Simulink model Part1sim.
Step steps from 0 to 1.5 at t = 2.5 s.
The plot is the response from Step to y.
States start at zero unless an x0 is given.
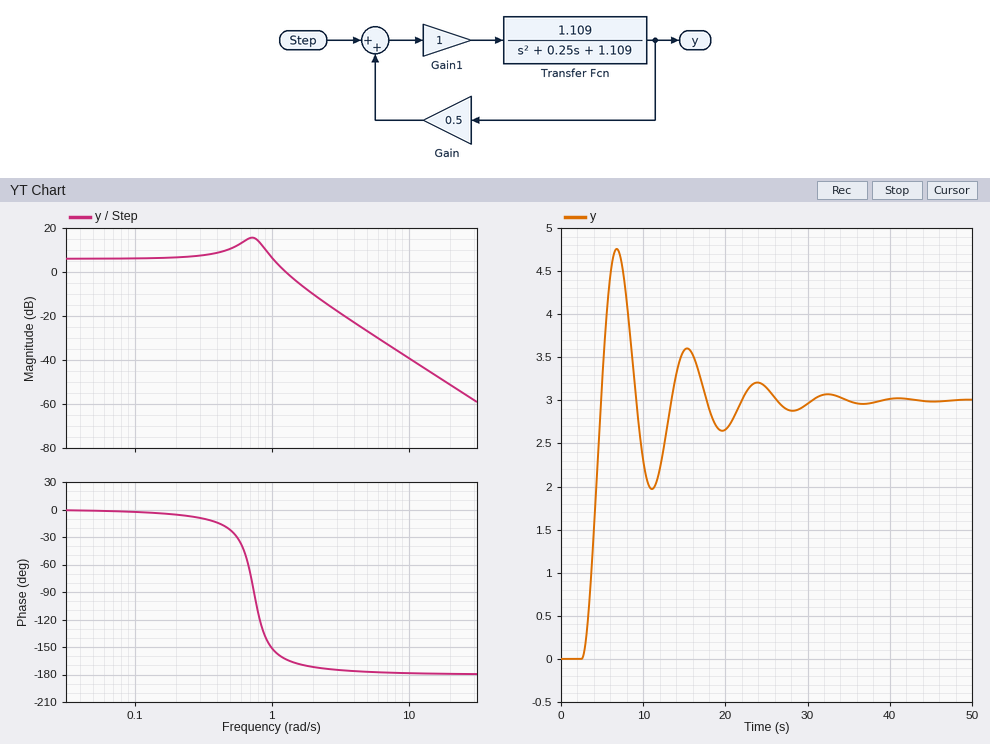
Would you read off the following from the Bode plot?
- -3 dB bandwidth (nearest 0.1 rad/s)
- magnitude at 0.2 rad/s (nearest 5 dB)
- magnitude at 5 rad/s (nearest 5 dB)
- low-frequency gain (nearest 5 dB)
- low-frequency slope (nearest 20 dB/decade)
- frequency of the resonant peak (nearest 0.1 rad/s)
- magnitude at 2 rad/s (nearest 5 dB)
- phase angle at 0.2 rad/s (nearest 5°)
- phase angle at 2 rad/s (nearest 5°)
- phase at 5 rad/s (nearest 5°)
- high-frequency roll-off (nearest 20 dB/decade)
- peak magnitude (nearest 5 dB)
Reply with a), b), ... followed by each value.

a) 1.1 rad/s
b) 5 dB
c) -25 dB
d) 5 dB
e) 0 dB/decade
f) 0.7 rad/s
g) -10 dB
h) -5°
i) -170°
j) -175°
k) -40 dB/decade
l) 15 dB
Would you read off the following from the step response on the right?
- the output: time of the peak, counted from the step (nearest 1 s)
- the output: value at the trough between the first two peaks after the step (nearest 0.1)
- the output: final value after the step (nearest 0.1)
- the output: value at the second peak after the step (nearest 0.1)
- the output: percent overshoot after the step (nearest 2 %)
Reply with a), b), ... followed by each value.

a) 4 s
b) 2.0
c) 3.0
d) 3.6
e) 58 %
